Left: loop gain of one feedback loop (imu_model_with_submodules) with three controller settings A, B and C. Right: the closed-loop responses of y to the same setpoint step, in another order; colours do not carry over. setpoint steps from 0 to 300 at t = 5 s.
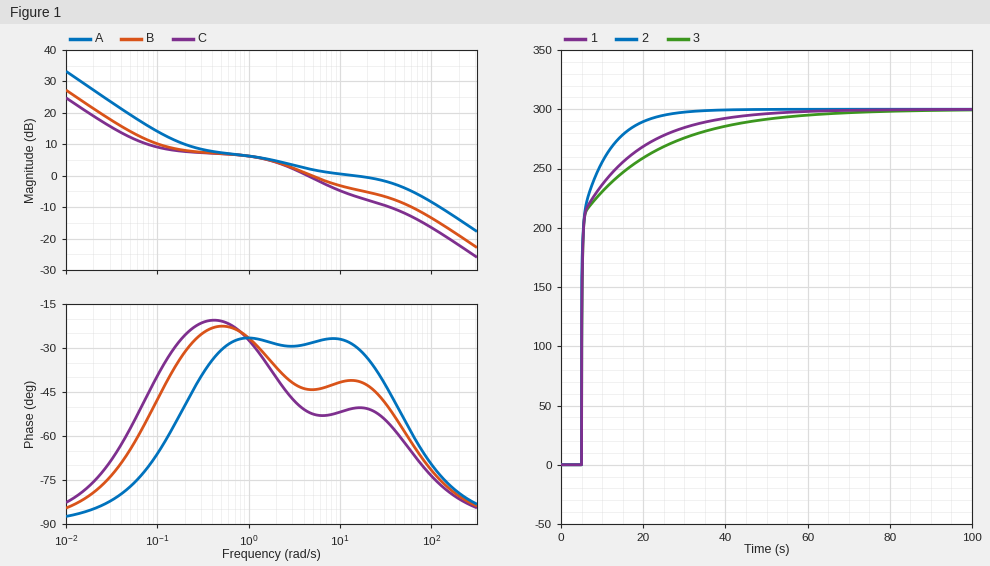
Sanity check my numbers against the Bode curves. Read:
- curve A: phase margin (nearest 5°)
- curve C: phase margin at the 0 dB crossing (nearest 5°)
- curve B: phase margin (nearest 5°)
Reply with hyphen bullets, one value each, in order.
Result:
- 150°
- 130°
- 135°
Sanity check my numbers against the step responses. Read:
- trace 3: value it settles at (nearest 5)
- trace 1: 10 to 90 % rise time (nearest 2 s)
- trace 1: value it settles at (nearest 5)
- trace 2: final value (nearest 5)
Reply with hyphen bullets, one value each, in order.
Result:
- 300
- 16 s
- 300
- 300
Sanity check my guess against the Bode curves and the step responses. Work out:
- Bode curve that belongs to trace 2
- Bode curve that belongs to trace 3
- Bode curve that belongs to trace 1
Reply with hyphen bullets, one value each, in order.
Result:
- A
- C
- B
